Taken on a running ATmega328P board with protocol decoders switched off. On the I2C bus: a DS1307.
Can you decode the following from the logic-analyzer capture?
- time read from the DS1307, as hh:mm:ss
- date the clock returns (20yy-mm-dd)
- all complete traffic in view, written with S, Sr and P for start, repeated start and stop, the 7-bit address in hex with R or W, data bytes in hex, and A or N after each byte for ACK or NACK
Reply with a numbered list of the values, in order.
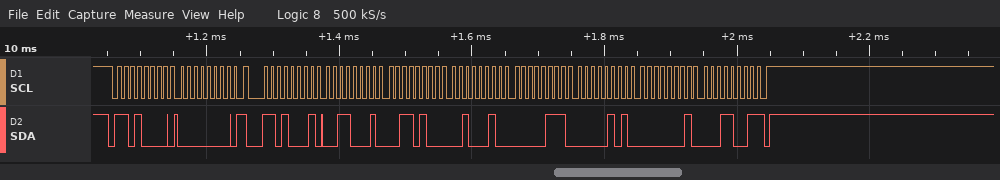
1. 22:34:31
2. 2019-01-05
3. S 68W A 00 A Sr 68R A 31 A 34 A 22 A 07 A 05 A 01 A 19 N P
